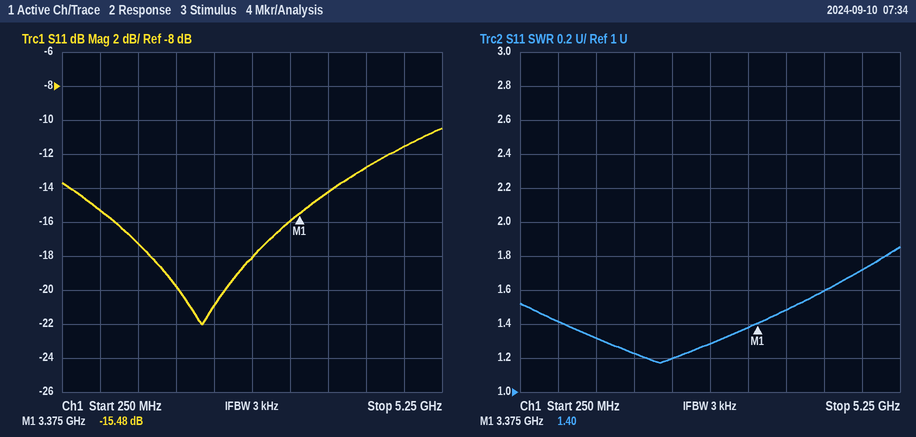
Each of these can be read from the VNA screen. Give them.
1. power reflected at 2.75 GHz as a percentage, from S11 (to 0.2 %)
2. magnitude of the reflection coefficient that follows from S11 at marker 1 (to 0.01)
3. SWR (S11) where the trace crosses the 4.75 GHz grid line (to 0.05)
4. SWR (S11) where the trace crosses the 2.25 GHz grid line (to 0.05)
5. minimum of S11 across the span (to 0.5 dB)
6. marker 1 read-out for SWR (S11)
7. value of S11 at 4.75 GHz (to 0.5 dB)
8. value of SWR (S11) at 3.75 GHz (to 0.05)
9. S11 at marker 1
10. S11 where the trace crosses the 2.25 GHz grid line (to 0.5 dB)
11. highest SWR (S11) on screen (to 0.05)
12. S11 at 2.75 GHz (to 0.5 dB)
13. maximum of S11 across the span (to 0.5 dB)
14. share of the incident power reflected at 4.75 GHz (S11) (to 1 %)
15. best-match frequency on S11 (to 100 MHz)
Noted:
1.6 %
0.17
1.70
1.20
-22.0 dB
1.40
-11.5 dB
1.50
-15.48 dB
-21.0 dB
1.85
-18.0 dB
-10.5 dB
7 %
2.1 GHz
